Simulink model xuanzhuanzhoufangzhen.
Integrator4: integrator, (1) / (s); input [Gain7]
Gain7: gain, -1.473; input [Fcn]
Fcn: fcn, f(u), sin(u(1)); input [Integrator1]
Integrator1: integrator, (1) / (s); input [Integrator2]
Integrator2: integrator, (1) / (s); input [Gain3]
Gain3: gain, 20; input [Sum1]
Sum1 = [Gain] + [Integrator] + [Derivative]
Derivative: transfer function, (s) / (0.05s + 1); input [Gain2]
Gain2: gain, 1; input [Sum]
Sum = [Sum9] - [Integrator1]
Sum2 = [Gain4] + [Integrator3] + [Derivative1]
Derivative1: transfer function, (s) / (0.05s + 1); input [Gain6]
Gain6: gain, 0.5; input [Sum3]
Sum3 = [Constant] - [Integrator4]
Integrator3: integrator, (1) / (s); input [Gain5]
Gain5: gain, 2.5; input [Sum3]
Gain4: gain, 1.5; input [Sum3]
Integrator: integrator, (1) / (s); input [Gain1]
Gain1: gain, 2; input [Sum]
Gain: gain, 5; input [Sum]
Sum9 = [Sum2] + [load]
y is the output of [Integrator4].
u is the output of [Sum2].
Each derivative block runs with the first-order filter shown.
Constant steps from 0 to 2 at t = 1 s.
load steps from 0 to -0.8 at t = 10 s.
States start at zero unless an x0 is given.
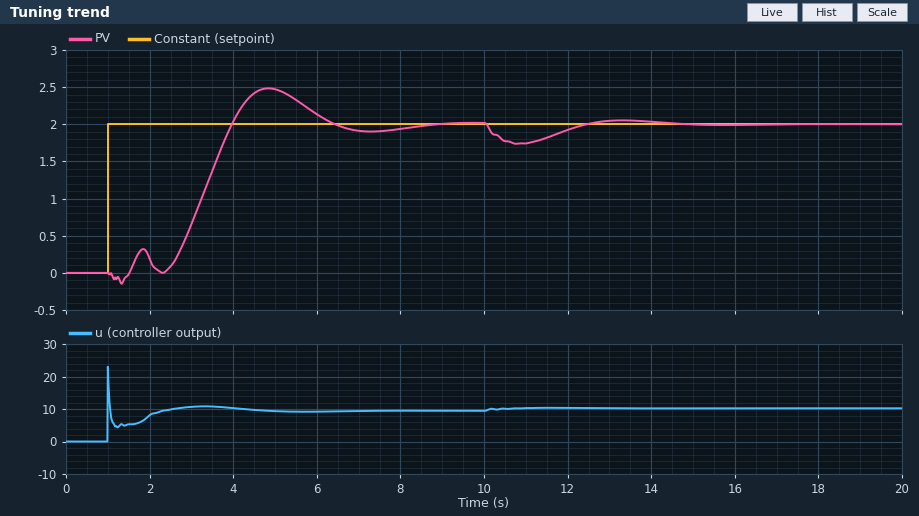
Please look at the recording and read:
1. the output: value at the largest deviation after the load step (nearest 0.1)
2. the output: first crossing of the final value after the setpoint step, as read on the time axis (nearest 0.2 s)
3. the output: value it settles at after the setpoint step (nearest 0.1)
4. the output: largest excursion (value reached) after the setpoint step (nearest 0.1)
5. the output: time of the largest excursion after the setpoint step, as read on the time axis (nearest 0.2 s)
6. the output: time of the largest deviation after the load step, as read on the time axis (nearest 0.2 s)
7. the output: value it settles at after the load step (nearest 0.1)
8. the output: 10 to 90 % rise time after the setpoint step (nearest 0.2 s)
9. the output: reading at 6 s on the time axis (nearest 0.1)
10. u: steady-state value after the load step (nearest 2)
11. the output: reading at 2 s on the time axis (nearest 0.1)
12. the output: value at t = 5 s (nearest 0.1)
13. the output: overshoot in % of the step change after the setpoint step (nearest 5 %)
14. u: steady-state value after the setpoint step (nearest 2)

1.7
4.0 s
2.0
2.5
4.8 s
10.8 s
2.0
2.2 s
2.1
10
0.2
2.5
25 %
10
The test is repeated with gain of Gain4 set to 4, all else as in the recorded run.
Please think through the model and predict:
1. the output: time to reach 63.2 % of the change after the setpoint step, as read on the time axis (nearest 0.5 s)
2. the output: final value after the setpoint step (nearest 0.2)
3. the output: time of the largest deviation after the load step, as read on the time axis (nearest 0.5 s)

3.0 s
2.0
10.5 s
